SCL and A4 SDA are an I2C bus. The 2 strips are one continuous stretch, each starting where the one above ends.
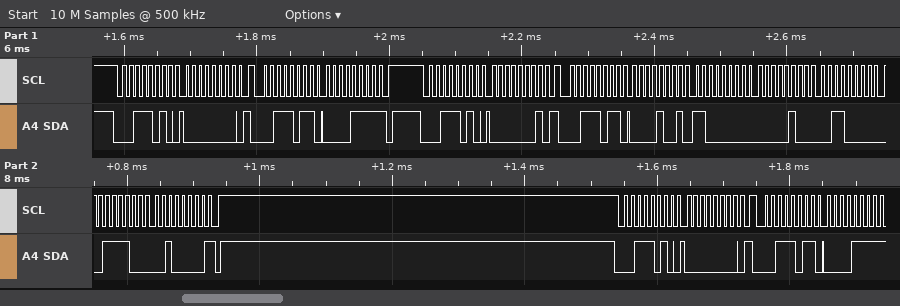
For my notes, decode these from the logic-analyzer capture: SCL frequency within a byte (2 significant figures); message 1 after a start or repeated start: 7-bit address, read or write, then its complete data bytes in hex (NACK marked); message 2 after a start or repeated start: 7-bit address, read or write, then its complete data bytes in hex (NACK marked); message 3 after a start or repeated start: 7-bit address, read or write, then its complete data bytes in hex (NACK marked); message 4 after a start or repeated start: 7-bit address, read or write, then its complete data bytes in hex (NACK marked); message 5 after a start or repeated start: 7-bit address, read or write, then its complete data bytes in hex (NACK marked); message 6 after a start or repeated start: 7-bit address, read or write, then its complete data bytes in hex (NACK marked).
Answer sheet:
100 kHz
0x1D write: 00
0x1D read: 0F NACK
0x1D write: 01
0x1D read: 09 C0 04 30 3C 20 NACK
0x1D write: 00
0x1D read: 0F NACK
